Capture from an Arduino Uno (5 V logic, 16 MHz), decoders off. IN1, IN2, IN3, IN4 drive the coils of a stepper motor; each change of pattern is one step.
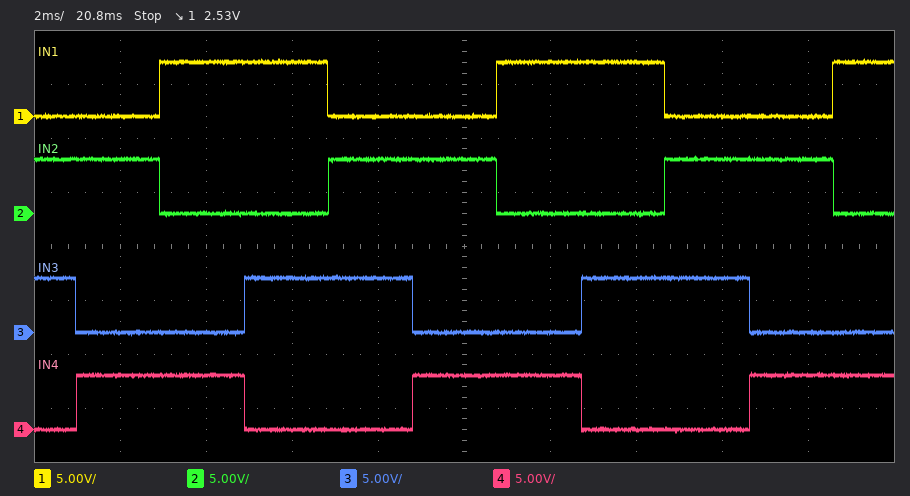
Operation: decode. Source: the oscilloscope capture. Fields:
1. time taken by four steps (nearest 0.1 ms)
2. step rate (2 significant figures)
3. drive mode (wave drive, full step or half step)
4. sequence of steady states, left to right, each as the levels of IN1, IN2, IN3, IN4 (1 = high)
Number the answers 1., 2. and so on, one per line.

1. 7.8 ms
2. 510 steps/s
3. full step
4. 0110 0101 1001 1010 0110 0101 1001 1010 0110 0101 1001
